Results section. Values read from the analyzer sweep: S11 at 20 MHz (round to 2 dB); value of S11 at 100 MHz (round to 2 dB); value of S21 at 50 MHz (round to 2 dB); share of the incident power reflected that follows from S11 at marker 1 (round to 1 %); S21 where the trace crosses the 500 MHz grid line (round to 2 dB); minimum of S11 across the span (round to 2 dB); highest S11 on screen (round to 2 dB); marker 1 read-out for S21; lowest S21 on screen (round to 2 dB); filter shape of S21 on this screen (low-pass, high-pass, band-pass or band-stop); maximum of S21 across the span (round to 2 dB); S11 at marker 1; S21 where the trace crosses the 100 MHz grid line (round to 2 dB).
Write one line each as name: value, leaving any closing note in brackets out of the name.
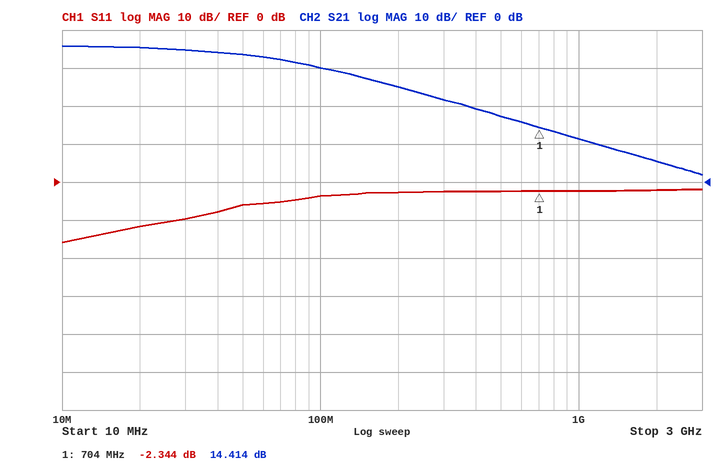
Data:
S11 at 20 MHz: -12 dB
value of S11 at 100 MHz: -4 dB
value of S21 at 50 MHz: 34 dB
share of the incident power reflected that follows from S11 at marker 1: 58 %
S21 where the trace crosses the 500 MHz grid line: 18 dB
minimum of S11 across the span: -16 dB
highest S11 on screen: -2 dB
marker 1 read-out for S21: 14.414 dB
lowest S21 on screen: 2 dB
filter shape of S21 on this screen: low-pass
maximum of S21 across the span: 36 dB
S11 at marker 1: -2.344 dB
S21 where the trace crosses the 100 MHz grid line: 30 dB
